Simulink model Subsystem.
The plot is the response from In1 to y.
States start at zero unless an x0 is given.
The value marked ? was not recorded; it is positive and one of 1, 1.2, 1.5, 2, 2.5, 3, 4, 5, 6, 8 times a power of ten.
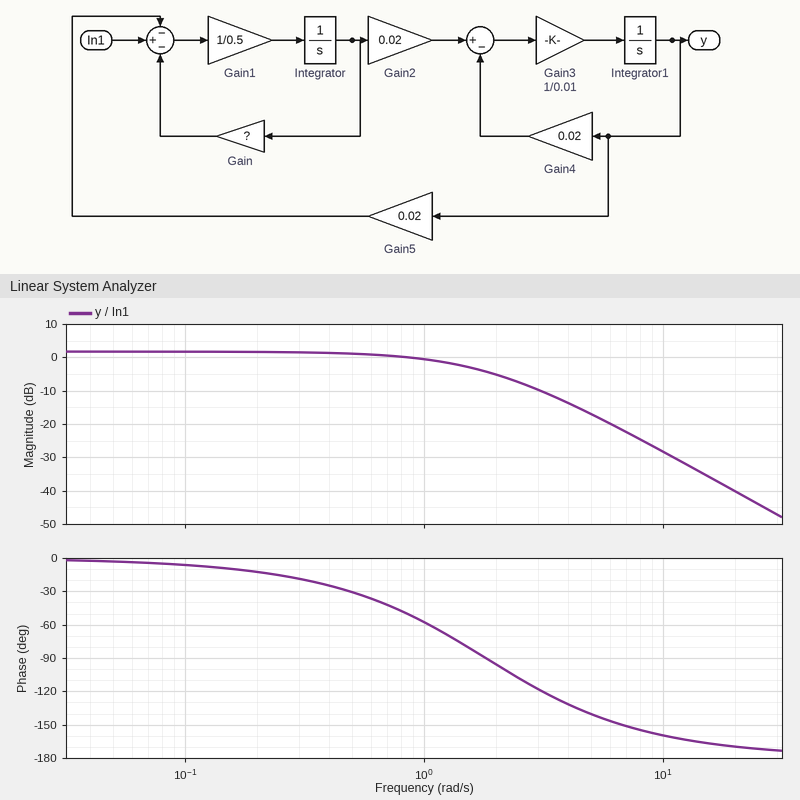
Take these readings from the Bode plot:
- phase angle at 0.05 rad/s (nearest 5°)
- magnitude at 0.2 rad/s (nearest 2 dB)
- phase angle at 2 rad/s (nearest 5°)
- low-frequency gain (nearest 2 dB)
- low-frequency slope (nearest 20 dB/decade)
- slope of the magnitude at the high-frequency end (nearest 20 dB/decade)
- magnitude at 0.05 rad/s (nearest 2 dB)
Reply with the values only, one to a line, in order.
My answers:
-5°
2 dB
-95°
2 dB
0 dB/decade
-40 dB/decade
2 dB
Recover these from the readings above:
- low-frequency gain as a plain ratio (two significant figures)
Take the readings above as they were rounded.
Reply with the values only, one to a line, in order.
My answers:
1.3
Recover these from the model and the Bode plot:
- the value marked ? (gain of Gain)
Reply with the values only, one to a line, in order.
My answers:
0.8
